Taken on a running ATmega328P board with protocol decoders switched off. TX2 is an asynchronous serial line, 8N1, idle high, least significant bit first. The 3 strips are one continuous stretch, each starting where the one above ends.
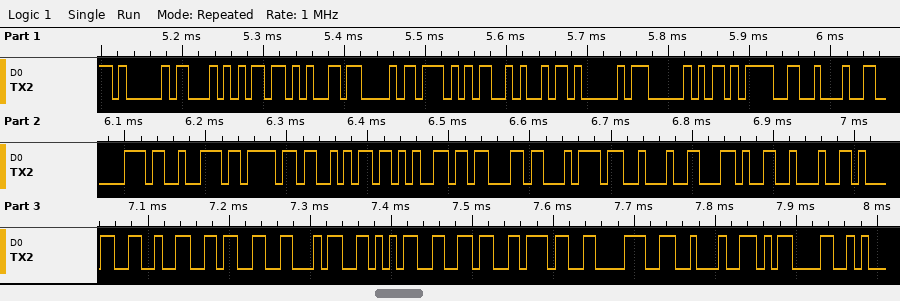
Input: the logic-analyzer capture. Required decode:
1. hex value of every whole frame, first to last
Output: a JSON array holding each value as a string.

["0x41 0x54 0x2B 0x43 0x57 0x4A 0x41 0x50 0x3D 0x22 0x70 0x72 0x6F 0x6A 0x65 0x63 0x74 0x22 0x2C 0x22 0x31 0x32 0x33 0x34 0x35 0x36 0x37 0x38 0x22 0x0D"]
